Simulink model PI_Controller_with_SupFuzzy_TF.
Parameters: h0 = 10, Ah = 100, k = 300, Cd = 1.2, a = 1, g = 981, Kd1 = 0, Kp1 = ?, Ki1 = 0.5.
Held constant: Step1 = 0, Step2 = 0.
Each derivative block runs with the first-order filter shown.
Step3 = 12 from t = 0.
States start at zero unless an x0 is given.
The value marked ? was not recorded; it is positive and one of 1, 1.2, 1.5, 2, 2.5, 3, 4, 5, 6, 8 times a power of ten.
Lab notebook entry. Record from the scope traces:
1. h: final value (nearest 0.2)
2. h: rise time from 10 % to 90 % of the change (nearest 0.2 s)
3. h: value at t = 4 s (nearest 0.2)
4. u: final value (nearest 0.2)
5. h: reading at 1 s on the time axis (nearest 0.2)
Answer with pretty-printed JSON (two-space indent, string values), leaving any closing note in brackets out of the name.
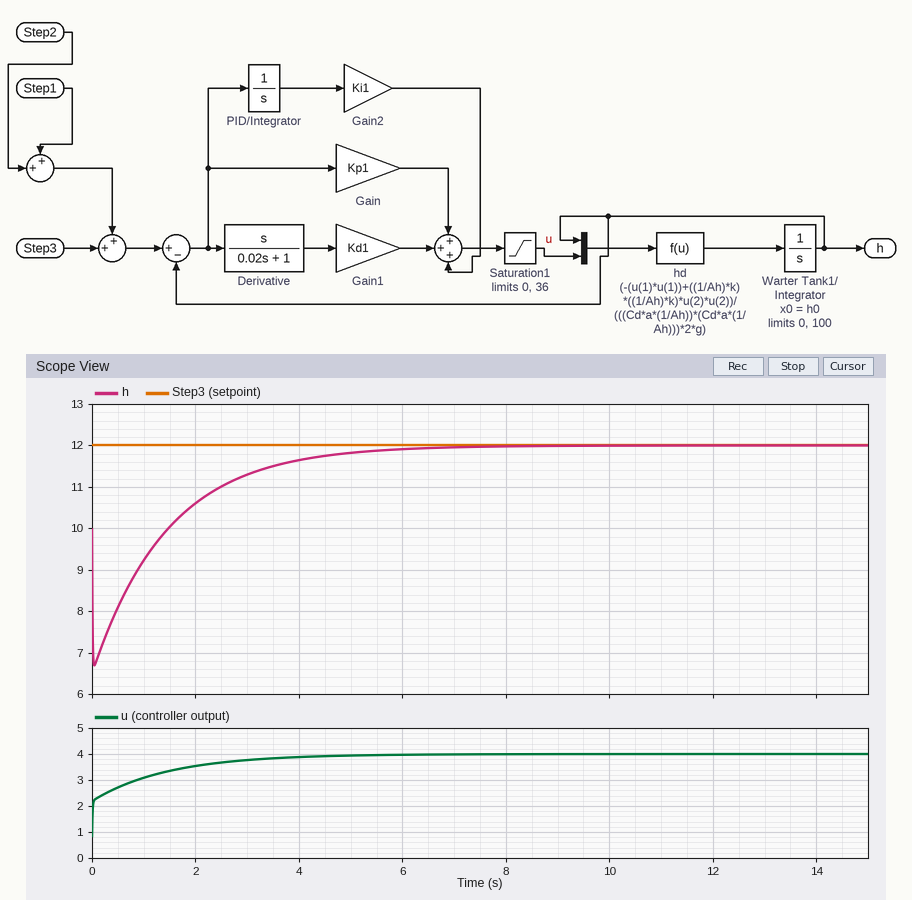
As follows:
{
  "h: final value": "12.0",
  "h: rise time from 10 % to 90 % of the change": "3.2 s",
  "h: value at t = 4 s": "11.6",
  "u: final value": "4.0",
  "h: reading at 1 s on the time axis": "9.2"
}
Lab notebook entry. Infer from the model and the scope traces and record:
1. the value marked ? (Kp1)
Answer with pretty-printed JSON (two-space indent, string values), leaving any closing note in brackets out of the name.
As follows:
{
  "the value marked ?": "0.4"
}
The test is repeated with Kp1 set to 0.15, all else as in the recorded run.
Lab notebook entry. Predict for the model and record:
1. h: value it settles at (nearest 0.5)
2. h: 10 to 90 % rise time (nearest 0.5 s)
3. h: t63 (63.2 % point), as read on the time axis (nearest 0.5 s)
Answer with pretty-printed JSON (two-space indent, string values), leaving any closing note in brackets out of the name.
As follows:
{
  "h: value it settles at": "12.0",
  "h: 10 to 90 % rise time": "2.0 s",
  "h: t63 (63.2 % point), as read on the time axis": "2.5 s"
}
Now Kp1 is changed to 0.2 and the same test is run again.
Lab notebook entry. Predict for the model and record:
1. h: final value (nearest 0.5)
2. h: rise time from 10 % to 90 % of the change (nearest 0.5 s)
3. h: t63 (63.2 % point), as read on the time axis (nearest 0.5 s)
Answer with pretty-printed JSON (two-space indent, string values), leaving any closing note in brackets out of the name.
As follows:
{
  "h: final value": "12.0",
  "h: rise time from 10 % to 90 % of the change": "2.5 s",
  "h: t63 (63.2 % point), as read on the time axis": "2.5 s"
}
